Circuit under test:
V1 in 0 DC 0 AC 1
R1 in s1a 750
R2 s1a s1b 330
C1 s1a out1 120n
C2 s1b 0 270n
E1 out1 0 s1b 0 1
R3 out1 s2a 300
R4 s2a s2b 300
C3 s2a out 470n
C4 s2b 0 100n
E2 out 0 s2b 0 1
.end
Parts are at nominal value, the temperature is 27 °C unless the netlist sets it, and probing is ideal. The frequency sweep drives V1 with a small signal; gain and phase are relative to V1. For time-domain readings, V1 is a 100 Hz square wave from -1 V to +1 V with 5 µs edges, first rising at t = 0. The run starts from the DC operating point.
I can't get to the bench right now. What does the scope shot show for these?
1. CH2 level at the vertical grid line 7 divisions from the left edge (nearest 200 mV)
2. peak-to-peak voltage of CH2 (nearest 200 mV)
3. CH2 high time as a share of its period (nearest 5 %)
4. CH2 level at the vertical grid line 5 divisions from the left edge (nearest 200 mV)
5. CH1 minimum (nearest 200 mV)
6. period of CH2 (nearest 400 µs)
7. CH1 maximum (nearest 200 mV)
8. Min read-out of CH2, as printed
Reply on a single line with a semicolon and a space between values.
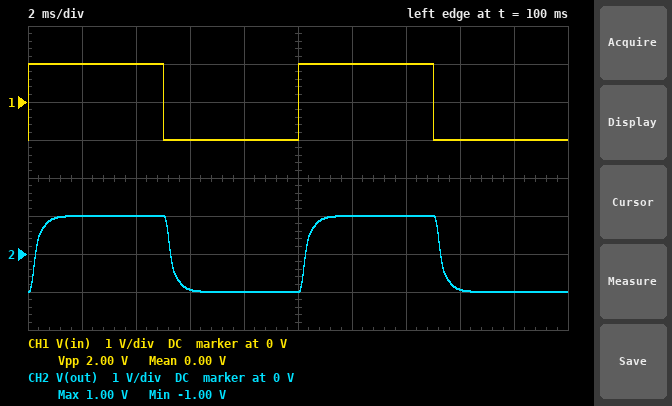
1.0 V; 2.0 V; 50 %; -1.0 V; -1.0 V; 10.0 ms; 1.0 V; -1.00 V
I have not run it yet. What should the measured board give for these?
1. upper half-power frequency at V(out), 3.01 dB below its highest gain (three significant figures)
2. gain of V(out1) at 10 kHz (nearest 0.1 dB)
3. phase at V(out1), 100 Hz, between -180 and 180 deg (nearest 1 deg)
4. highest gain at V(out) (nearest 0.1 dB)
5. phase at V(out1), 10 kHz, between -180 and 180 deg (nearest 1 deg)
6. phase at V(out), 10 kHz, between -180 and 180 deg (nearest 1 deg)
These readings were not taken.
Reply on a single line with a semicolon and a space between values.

649 Hz; -31.1 dB; -10 deg; 0 dB; -149 deg; 44 deg
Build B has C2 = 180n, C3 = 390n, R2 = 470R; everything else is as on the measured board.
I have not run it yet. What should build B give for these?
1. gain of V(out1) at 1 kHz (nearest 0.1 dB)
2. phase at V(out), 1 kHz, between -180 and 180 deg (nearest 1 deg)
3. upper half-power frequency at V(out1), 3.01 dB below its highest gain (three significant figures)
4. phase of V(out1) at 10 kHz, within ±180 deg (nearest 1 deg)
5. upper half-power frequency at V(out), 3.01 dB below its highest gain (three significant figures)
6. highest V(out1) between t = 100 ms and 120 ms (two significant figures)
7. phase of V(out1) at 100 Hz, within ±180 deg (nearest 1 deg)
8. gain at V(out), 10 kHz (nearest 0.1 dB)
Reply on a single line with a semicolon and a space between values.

-3.8 dB; -87 deg; 855 Hz; -155 deg; 945 Hz; 1.0 V; -8 deg; -52.7 dB
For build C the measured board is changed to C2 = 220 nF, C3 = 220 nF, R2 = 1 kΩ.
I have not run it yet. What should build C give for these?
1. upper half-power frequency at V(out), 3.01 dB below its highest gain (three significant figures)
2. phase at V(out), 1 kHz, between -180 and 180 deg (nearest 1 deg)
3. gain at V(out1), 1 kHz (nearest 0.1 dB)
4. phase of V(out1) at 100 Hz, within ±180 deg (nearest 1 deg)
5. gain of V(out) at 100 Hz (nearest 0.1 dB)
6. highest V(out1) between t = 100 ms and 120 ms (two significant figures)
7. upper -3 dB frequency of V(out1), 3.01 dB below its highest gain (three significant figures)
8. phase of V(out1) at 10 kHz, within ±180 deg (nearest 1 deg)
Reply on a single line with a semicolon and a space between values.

477 Hz; -107 deg; -7.7 dB; -14 deg; -0.2 dB; 1.0 V; 475 Hz; -163 deg
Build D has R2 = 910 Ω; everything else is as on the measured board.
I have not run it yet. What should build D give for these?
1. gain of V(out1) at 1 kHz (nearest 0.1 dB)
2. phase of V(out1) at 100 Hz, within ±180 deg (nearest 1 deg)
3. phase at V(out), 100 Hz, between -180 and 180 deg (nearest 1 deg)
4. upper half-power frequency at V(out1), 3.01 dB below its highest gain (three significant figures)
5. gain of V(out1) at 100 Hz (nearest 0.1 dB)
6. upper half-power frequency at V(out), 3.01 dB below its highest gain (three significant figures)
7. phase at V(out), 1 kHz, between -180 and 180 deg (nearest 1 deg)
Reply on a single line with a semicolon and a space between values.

-9.0 dB; -16 deg; -18 deg; 398 Hz; -0.3 dB; 411 Hz; -112 deg
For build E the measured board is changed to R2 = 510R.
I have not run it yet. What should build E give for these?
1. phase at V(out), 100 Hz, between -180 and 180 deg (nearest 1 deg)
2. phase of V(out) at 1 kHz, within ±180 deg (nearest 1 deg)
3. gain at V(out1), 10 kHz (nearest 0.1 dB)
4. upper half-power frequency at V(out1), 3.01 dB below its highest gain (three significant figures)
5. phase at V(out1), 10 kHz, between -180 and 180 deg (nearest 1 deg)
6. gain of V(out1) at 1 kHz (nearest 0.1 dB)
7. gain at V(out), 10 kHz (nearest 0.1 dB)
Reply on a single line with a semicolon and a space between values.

-14 deg; -101 deg; -34.4 dB; 523 Hz; -156 deg; -6.8 dB; -58.6 dB
